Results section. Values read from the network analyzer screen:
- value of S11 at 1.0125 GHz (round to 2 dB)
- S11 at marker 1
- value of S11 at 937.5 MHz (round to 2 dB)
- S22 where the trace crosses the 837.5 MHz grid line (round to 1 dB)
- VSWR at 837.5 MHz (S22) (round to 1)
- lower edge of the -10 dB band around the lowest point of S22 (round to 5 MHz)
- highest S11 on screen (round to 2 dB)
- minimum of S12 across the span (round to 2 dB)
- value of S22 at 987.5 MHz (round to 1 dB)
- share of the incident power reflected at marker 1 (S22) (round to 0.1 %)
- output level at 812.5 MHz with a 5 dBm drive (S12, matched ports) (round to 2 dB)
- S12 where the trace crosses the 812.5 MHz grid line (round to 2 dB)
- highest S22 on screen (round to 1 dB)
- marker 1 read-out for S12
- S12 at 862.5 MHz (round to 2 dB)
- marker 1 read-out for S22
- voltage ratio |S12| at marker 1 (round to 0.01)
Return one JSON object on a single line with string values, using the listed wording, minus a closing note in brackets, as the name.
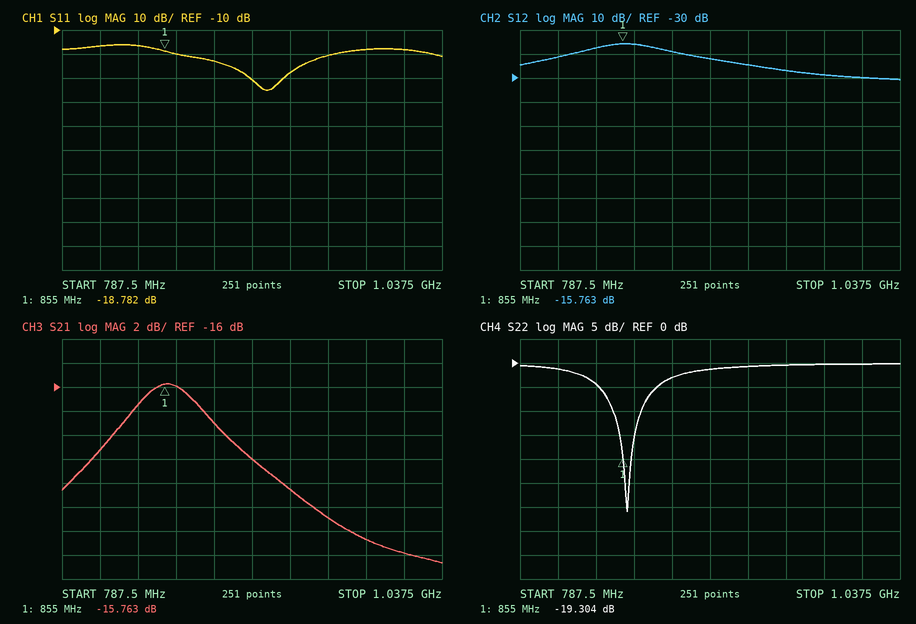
{"value of S11 at 1.0125 GHz": "-18 dB", "S11 at marker 1": "-18.782 dB", "value of S11 at 937.5 MHz": "-28 dB", "S22 where the trace crosses the 837.5 MHz grid line": "-4 dB", "VSWR at 837.5 MHz (S22)": "4", "lower edge of the -10 dB band around the lowest point of S22": "850 MHz", "highest S11 on screen": "-16 dB", "minimum of S12 across the span": "-30 dB", "value of S22 at 987.5 MHz": "0 dB", "share of the incident power reflected at marker 1 (S22)": "1.2 %", "output level at 812.5 MHz with a 5 dBm drive (S12, matched ports)": "-16 dBm", "S12 where the trace crosses the 812.5 MHz grid line": "-22 dB", "highest S22 on screen": "0 dB", "marker 1 read-out for S12": "-15.763 dB", "S12 at 862.5 MHz": "-16 dB", "marker 1 read-out for S22": "-19.304 dB", "voltage ratio |S12| at marker 1": "0.16"}
